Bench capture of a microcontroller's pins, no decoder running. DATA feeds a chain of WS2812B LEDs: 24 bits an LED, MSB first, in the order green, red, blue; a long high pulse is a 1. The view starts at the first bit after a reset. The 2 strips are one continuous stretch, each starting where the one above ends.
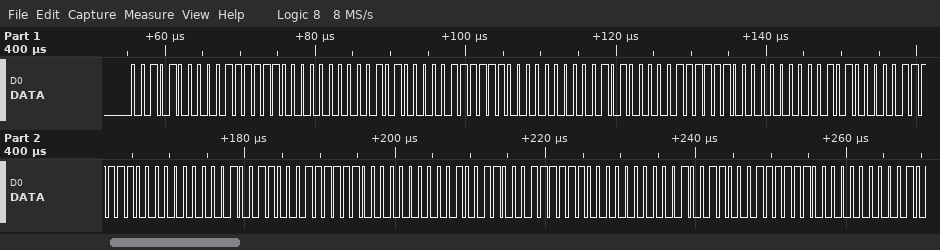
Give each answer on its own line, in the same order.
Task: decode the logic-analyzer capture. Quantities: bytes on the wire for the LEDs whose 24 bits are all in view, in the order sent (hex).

28 3F 00 28 3F 00 28 3F 00 28 3F 00 26 3F 00 26 3F 00 26 3F 00
